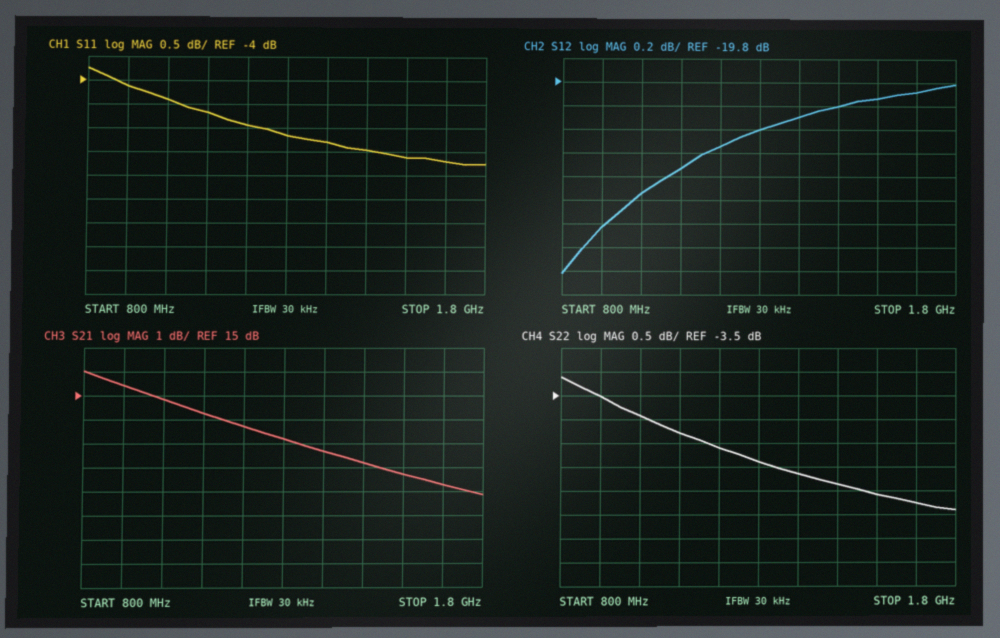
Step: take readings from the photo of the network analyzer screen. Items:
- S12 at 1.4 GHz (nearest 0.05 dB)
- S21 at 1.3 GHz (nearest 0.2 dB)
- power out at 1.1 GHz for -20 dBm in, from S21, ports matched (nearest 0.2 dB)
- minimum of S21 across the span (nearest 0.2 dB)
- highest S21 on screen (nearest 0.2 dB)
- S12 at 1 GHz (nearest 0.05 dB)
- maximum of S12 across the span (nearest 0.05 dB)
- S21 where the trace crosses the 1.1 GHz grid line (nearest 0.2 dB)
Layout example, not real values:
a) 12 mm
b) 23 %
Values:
a) -20.10 dB
b) 13.2 dB
c) -5.8 dBm
d) 10.8 dB
e) 16.0 dB
f) -20.75 dB
g) -19.80 dB
h) 14.2 dB
